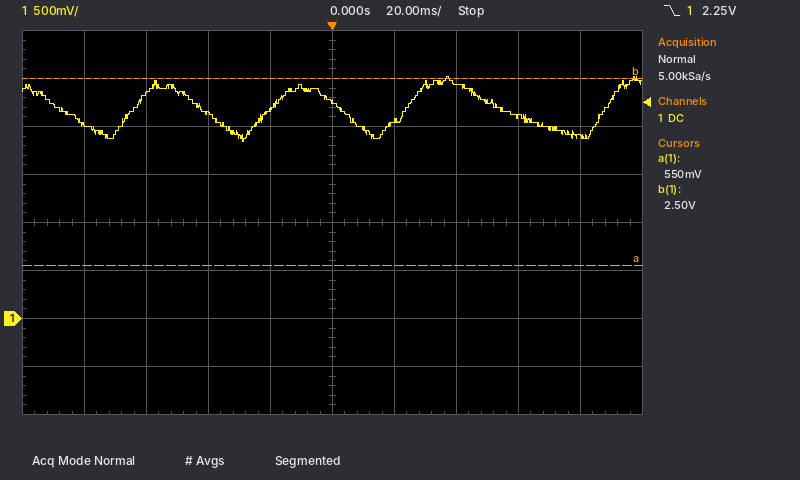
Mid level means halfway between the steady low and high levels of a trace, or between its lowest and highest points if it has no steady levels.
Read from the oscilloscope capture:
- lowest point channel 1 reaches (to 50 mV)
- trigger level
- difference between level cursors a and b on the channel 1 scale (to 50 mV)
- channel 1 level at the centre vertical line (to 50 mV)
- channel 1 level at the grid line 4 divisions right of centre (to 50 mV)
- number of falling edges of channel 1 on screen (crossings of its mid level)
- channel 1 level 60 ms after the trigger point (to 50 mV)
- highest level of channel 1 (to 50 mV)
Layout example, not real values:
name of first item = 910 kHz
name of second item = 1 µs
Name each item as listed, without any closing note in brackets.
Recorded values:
lowest point channel 1 reaches = 1.85 V
trigger level = 2.25 V
difference between level cursors a and b on the channel 1 scale = 1.95 V
channel 1 level at the centre vertical line = 2.25 V
channel 1 level at the grid line 4 divisions right of centre = 1.90 V
number of falling edges of channel 1 on screen = 4
channel 1 level 60 ms after the trigger point = 2.10 V
highest level of channel 1 = 2.50 V
